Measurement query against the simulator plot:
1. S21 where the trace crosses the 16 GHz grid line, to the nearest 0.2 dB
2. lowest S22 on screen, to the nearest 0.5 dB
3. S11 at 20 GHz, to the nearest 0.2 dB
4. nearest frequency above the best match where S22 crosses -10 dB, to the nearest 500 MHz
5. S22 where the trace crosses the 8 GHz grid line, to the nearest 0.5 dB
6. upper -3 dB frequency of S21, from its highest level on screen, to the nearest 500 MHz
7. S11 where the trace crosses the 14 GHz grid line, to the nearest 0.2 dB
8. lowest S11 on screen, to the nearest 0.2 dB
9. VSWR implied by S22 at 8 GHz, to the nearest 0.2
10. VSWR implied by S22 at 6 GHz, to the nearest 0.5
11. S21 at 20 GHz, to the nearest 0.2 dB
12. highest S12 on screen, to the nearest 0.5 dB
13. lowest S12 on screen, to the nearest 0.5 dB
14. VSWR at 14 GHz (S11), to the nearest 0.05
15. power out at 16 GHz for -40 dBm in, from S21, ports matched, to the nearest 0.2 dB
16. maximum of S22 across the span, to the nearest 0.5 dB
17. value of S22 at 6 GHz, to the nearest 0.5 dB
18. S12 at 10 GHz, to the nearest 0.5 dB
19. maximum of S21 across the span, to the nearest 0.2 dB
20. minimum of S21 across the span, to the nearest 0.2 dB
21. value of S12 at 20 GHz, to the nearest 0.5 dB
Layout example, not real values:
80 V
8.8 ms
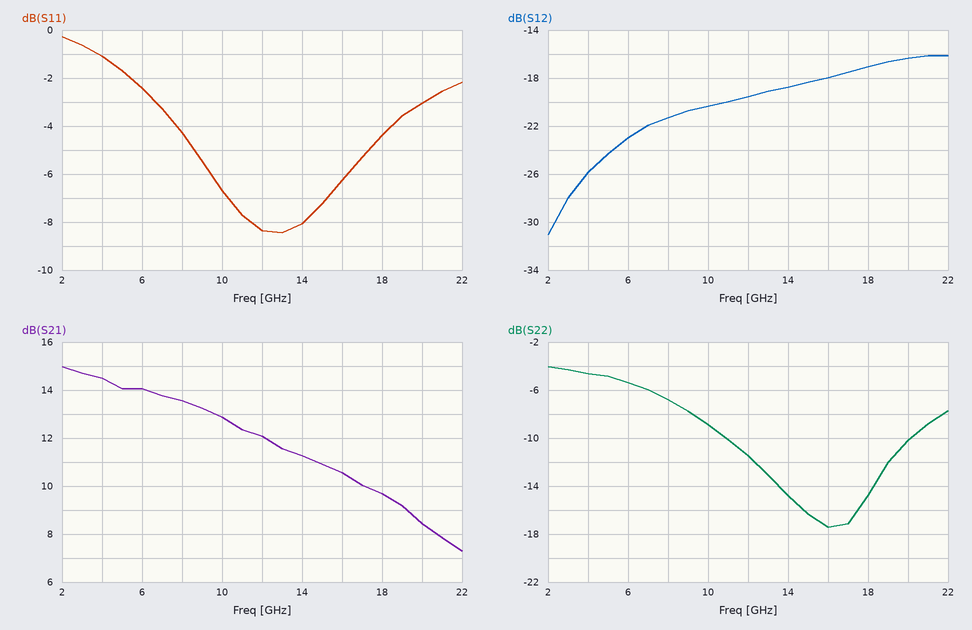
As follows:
10.6 dB
-17.5 dB
-3.0 dB
20.0 GHz
-7.0 dB
12.0 GHz
-8.0 dB
-8.4 dB
2.6
3.5
8.4 dB
-16.0 dB
-31.0 dB
2.30
-29.4 dBm
-4.0 dB
-5.5 dB
-20.5 dB
15.0 dB
7.2 dB
-16.5 dB
